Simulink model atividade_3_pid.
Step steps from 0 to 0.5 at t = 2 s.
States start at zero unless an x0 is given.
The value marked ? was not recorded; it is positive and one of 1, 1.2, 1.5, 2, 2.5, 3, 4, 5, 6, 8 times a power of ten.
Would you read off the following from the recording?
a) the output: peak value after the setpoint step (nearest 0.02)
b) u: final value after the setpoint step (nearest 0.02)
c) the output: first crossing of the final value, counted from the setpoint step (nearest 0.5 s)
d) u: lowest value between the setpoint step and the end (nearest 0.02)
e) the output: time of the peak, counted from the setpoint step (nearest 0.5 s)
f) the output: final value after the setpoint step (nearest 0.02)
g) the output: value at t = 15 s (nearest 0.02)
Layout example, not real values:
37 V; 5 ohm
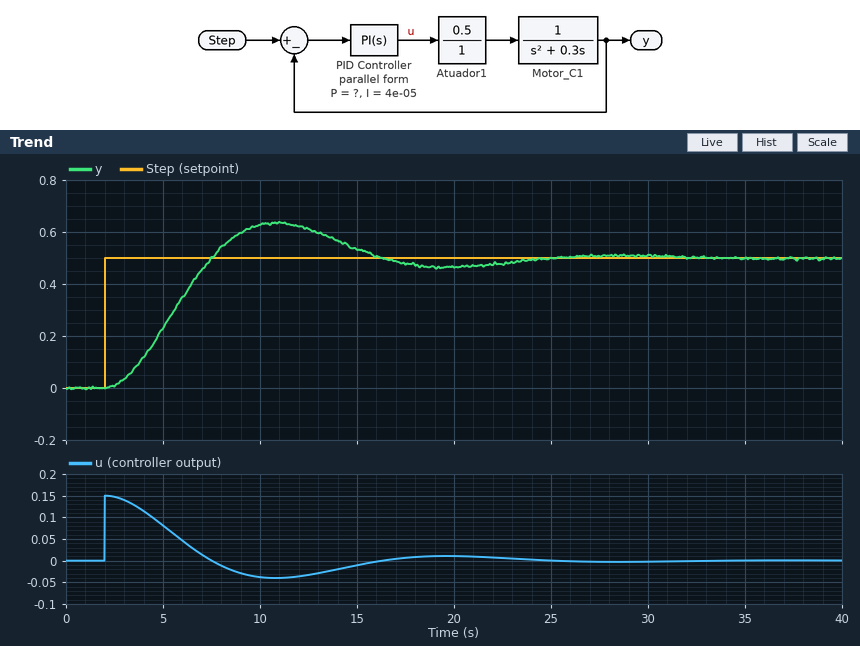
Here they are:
0.64; 0.00; 5.5 s; -0.04; 9.0 s; 0.50; 0.54
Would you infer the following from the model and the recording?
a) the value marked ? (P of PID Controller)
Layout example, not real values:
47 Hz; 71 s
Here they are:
0.3
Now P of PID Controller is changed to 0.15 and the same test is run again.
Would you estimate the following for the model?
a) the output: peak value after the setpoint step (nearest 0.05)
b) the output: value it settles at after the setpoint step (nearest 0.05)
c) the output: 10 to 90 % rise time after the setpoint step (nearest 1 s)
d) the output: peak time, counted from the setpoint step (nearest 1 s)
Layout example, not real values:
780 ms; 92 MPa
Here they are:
0.55; 0.50; 6 s; 14 s
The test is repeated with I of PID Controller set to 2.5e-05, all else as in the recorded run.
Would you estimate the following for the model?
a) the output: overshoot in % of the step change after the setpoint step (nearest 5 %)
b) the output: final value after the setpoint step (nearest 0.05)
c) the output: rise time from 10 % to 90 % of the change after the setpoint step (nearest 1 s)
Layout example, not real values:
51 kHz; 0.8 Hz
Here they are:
25 %; 0.50; 4 s
